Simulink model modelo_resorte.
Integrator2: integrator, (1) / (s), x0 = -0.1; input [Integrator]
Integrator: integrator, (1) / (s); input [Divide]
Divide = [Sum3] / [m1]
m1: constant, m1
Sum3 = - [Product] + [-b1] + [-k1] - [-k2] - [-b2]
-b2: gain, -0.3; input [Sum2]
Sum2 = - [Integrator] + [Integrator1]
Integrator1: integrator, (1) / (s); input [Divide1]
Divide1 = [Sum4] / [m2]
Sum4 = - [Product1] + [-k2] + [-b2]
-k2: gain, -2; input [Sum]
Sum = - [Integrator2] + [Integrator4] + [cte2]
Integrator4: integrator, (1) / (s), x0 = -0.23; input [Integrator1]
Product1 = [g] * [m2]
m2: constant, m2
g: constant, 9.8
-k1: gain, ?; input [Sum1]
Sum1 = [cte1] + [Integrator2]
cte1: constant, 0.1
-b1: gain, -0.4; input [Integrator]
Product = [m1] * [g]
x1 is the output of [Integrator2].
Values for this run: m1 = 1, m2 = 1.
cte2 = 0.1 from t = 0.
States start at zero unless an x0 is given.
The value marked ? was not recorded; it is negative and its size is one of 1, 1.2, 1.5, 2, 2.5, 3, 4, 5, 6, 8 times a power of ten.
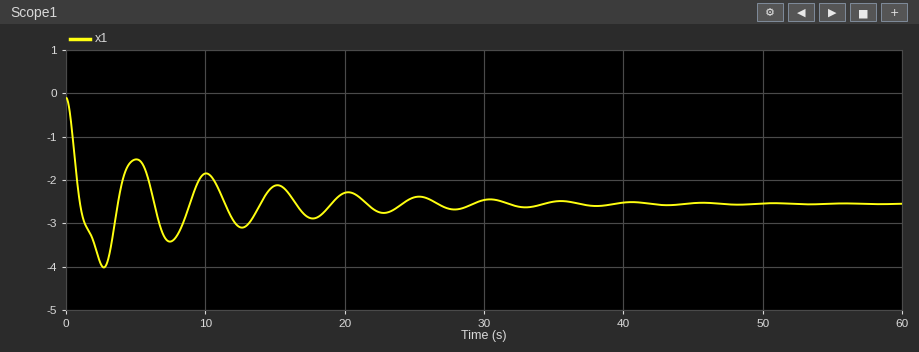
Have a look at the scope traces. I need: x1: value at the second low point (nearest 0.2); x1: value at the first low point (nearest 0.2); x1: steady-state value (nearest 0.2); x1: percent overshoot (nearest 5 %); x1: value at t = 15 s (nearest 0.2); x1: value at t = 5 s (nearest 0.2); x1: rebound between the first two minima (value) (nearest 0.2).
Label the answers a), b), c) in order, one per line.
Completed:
a) -3.4
b) -4.0
c) -2.6
d) 60 %
e) -2.2
f) -1.6
g) -1.6
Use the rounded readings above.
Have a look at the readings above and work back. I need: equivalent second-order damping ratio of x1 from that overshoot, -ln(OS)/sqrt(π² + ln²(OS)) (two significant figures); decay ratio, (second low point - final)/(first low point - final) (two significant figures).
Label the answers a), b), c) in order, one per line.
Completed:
a) 0.16
b) 0.57
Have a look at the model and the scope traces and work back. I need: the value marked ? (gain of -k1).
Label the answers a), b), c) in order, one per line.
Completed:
a) -8
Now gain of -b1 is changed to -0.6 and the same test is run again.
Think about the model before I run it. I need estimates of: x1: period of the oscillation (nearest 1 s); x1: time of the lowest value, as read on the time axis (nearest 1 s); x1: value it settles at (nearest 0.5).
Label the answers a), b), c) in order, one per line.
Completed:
a) 5 s
b) 3 s
c) -2.5
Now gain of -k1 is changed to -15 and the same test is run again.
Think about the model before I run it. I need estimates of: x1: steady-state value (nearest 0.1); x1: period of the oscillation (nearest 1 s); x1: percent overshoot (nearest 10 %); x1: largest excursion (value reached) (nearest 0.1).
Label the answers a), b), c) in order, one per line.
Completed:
a) -1.4
b) 5 s
c) 60 %
d) -2.2
